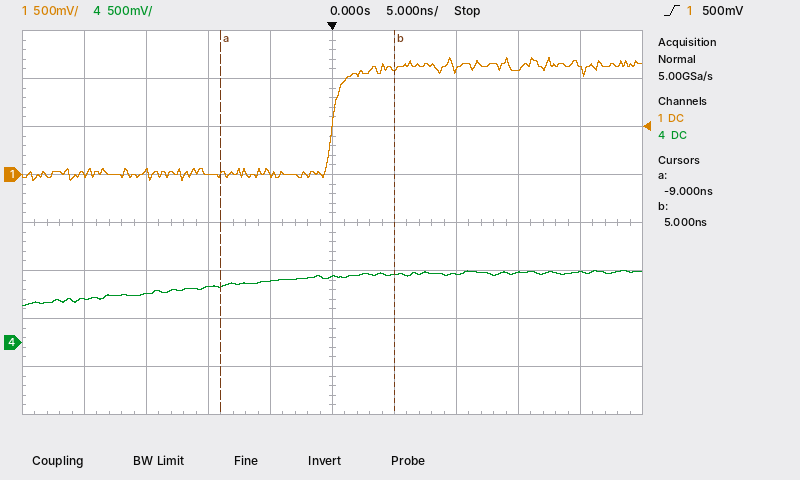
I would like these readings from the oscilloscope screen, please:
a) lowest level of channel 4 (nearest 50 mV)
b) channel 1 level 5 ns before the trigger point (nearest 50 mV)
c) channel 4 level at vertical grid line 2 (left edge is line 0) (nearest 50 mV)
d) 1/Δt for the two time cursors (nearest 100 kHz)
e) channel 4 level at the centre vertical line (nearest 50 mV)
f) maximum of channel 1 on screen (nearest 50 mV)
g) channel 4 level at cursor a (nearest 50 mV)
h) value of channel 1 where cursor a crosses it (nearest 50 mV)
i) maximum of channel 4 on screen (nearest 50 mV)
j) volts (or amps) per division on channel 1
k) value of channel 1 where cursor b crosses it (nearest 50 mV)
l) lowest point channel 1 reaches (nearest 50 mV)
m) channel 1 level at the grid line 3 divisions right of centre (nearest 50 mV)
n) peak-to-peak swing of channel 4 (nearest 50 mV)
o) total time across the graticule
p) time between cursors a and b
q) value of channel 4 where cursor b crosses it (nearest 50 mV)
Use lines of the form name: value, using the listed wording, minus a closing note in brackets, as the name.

lowest level of channel 4: 400 mV
channel 1 level 5 ns before the trigger point: 0 mV
channel 4 level at vertical grid line 2 (left edge is line 0): 500 mV
1/Δt for the two time cursors: 71.4 MHz
channel 4 level at the centre vertical line: 700 mV
maximum of channel 1 on screen: 1.20 V
channel 4 level at cursor a: 600 mV
value of channel 1 where cursor a crosses it: 0 mV
maximum of channel 4 on screen: 750 mV
volts (or amps) per division on channel 1: 500 mV
value of channel 1 where cursor b crosses it: 1.10 V
lowest point channel 1 reaches: -50 mV
channel 1 level at the grid line 3 divisions right of centre: 1.10 V
peak-to-peak swing of channel 4: 350 mV
total time across the graticule: 50 ns
time between cursors a and b: 14.0 ns
value of channel 4 where cursor b crosses it: 700 mV
